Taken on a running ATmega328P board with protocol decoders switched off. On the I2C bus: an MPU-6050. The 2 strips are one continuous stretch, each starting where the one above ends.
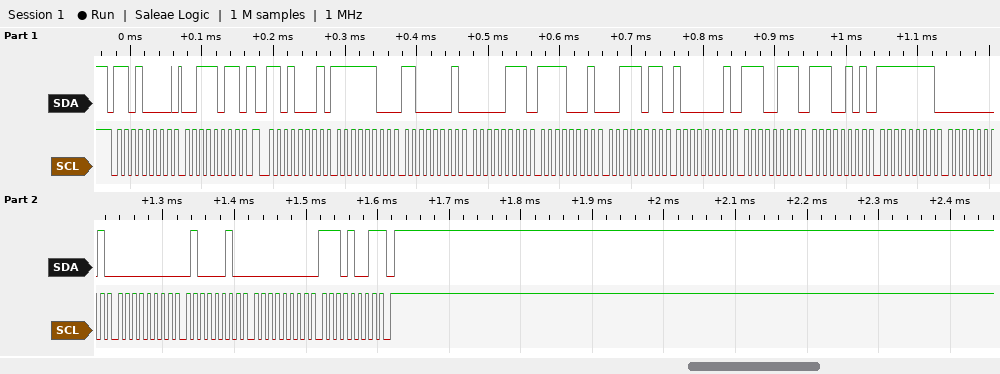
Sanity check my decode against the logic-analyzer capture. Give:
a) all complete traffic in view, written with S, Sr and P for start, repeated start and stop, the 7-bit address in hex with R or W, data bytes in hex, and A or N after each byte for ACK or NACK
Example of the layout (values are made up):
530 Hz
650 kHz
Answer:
S 68W A 3B A Sr 68R A FC A C1 A 07 A F1 A 3B A 81 A E7 A E5 A FF A 01 A 00 A 42 A 00 A E9 N P
